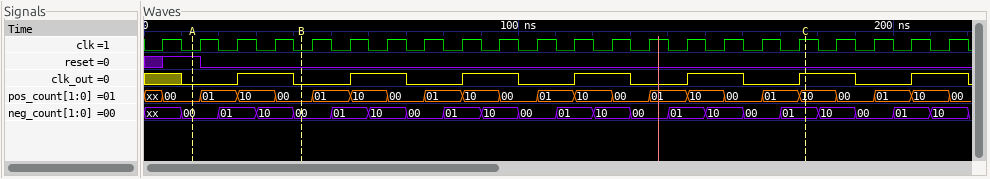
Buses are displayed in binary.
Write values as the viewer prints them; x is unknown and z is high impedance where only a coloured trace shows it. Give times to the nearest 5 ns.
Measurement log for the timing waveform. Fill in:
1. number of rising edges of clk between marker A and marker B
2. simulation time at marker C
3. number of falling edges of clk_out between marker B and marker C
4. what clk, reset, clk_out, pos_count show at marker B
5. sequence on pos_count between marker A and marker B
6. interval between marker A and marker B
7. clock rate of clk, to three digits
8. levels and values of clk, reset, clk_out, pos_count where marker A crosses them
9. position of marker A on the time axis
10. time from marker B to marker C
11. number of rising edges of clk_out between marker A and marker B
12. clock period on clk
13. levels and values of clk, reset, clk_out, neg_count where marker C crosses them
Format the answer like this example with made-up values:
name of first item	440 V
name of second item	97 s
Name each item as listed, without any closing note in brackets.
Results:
number of rising edges of clk between marker A and marker B	3
simulation time at marker C	175 ns
number of falling edges of clk_out between marker B and marker C	4
what clk, reset, clk_out, pos_count show at marker B	clk=0, reset=0, clk_out=0, pos_count=00
sequence on pos_count between marker A and marker B	00, 01, 10, 00
interval between marker A and marker B	30 ns
clock rate of clk, to three digits	100 MHz
levels and values of clk, reset, clk_out, pos_count where marker A crosses them	clk=0, reset=1, clk_out=0, pos_count=00
position of marker A on the time axis	15 ns
time from marker B to marker C	135 ns
number of rising edges of clk_out between marker A and marker B	1
clock period on clk	10 ns
levels and values of clk, reset, clk_out, neg_count where marker C crosses them	clk=1, reset=0, clk_out=1, neg_count=01
